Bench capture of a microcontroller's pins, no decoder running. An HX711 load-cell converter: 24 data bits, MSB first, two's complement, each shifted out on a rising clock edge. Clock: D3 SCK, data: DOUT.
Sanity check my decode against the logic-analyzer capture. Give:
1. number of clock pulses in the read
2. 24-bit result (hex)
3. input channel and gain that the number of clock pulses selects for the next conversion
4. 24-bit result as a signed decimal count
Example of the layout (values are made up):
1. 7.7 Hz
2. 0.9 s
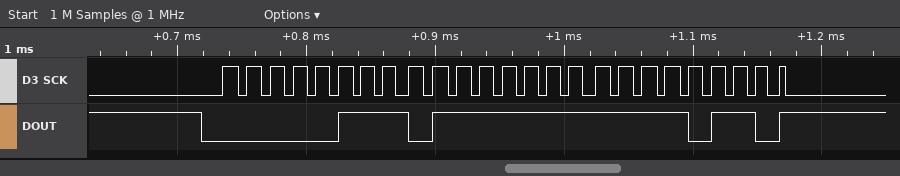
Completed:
1. 25
2. 0x077FF6
3. channel A, gain 128
4. 491510
